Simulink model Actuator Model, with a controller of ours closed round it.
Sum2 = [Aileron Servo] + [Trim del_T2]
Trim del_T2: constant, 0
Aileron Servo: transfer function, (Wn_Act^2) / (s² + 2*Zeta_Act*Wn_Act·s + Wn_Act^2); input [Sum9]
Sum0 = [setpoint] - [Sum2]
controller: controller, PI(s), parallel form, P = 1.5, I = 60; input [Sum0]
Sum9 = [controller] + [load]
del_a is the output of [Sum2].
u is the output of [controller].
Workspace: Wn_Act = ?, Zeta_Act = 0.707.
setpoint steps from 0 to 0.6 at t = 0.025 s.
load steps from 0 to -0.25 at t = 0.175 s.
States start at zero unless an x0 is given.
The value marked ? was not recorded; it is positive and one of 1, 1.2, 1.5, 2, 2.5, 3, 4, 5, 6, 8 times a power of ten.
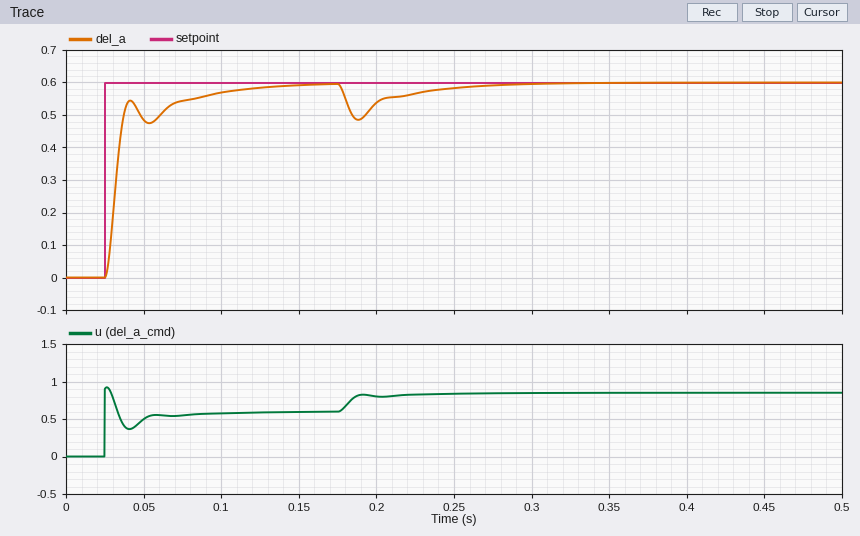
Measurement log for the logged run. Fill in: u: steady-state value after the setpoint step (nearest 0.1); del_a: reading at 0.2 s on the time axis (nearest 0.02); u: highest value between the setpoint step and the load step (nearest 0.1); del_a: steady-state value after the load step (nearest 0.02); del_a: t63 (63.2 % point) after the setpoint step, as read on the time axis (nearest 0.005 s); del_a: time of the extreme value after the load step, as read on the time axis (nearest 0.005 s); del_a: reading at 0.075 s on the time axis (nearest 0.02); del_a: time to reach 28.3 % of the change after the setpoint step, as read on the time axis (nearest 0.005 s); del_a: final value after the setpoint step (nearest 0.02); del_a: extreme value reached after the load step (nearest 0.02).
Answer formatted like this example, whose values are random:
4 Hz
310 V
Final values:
0.6
0.54
0.9
0.60
0.035 s
0.190 s
0.54
0.030 s
0.60
0.48
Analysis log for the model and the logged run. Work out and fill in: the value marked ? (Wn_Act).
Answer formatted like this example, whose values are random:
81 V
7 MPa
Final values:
150
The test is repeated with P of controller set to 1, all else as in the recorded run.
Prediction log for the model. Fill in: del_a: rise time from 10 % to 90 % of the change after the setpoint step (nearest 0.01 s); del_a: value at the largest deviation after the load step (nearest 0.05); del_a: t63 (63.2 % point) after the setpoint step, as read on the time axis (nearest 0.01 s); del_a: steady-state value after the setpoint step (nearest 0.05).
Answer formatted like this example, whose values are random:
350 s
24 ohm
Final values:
0.04 s
0.45
0.04 s
0.60
